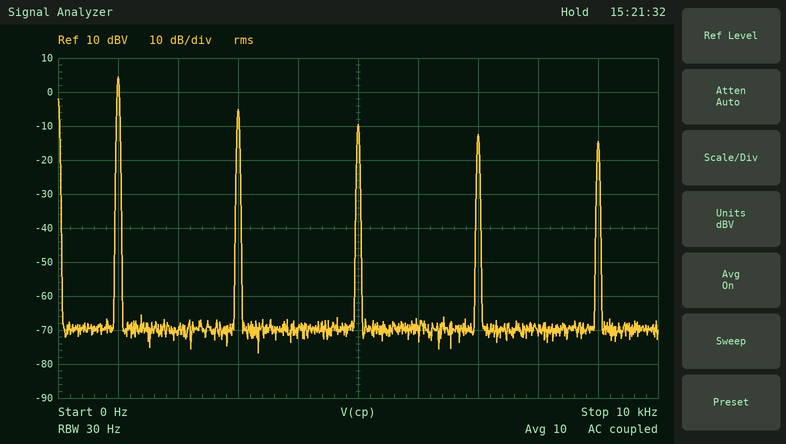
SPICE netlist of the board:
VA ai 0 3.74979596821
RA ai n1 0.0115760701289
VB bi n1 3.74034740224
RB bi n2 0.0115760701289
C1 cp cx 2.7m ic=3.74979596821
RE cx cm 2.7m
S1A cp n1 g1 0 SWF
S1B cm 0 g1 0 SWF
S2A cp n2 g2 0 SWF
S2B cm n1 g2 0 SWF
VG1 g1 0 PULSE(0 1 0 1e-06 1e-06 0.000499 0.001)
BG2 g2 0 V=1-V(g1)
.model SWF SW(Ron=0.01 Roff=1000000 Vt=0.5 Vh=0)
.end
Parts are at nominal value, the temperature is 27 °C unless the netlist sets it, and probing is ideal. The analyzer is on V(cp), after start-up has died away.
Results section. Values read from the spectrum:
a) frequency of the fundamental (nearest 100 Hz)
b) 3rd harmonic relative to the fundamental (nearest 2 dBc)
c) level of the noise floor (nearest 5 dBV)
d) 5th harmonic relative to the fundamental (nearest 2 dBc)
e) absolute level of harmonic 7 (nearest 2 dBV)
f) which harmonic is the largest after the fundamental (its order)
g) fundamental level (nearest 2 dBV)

1.0 kHz
-10 dBc
-70 dBV
-14 dBc
-12 dBV
3
4 dBV
